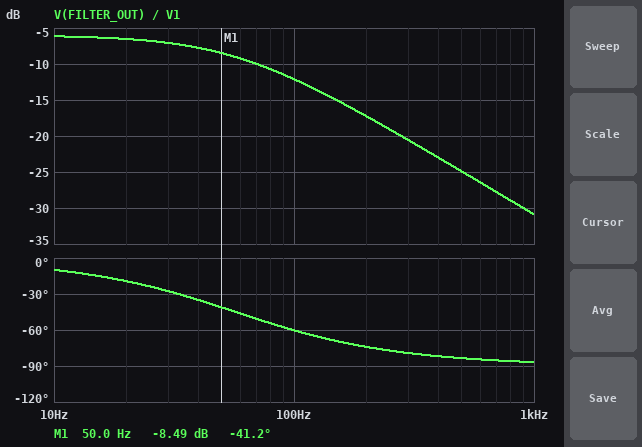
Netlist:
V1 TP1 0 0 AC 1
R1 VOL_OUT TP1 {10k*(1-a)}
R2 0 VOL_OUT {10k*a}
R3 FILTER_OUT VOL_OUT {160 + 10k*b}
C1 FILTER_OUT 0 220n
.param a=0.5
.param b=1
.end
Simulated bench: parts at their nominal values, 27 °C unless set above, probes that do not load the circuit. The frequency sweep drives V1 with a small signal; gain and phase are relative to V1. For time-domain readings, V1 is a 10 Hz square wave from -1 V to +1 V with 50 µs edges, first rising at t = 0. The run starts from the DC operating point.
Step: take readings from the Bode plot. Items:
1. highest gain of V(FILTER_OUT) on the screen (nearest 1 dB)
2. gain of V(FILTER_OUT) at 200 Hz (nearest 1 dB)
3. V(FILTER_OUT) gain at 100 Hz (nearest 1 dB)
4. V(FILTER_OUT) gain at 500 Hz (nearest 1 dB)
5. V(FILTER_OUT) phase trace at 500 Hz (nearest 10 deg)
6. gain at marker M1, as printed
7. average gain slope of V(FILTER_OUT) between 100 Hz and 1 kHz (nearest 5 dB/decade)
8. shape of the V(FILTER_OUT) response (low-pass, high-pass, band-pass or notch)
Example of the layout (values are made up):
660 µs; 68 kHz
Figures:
-6 dB; -17 dB; -12 dB; -25 dB; -80 deg; -8.49 dB; -20 dB/decade; low-pass
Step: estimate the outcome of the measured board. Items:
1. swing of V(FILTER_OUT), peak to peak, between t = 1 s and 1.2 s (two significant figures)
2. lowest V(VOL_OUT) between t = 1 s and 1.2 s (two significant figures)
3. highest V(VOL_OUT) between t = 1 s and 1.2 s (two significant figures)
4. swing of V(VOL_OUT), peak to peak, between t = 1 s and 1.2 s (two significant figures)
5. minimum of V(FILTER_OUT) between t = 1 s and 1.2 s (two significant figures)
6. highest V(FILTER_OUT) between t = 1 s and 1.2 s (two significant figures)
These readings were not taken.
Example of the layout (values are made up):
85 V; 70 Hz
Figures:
1.0 V; -500 mV; 500 mV; 1.0 V; -500 mV; 500 mV
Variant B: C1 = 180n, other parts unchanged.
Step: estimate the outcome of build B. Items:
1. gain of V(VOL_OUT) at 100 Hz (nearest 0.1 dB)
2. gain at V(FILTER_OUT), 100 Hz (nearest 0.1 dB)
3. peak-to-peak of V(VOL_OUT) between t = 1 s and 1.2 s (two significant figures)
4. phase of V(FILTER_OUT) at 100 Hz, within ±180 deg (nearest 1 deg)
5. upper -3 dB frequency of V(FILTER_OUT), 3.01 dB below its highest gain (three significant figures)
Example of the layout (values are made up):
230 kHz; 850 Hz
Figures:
-7.2 dB; -10.9 dB; 1.0 V; -55 deg; 69.8 Hz
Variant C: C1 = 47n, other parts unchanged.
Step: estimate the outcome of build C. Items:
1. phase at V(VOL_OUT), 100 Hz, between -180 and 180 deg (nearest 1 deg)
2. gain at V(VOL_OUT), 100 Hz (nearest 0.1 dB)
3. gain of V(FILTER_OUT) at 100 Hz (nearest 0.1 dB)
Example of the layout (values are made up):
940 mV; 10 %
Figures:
-4 deg; -6.2 dB; -6.6 dB
